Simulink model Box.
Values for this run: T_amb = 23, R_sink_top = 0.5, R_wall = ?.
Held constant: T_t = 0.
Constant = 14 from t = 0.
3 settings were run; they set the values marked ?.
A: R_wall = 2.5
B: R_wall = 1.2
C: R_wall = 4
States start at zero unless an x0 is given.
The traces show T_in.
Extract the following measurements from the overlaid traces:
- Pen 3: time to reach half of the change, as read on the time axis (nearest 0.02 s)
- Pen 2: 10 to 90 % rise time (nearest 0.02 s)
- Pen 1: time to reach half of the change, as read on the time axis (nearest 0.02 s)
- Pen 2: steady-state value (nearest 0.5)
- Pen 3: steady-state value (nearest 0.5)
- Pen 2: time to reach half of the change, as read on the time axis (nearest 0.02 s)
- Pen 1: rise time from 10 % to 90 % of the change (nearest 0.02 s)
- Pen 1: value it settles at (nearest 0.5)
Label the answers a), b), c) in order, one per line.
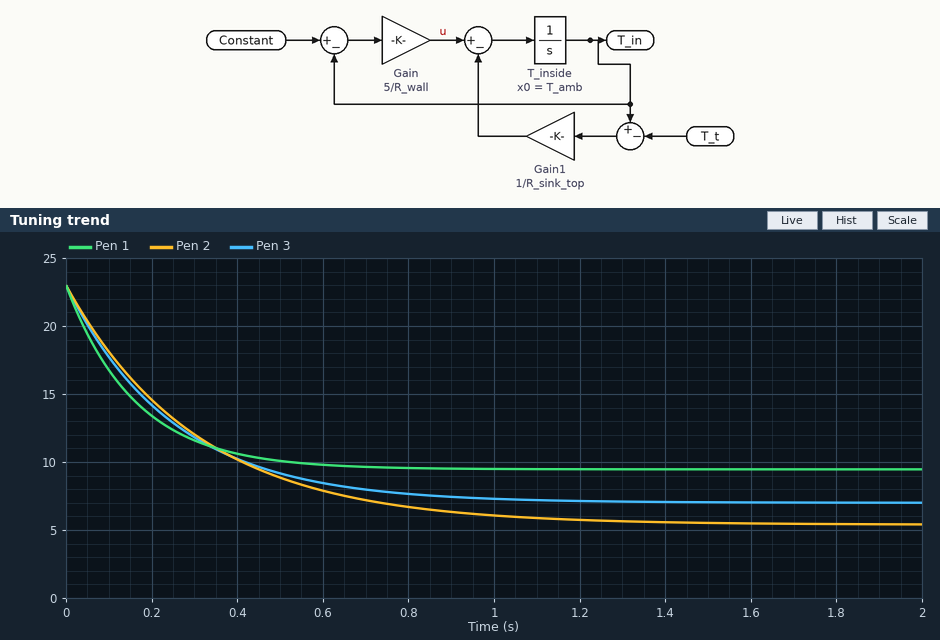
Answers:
a) 0.18 s
b) 0.68 s
c) 0.12 s
d) 5.5
e) 7.0
f) 0.22 s
g) 0.36 s
h) 9.5
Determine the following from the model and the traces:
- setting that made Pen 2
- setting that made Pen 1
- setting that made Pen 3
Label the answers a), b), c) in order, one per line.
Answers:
a) C
b) B
c) A
